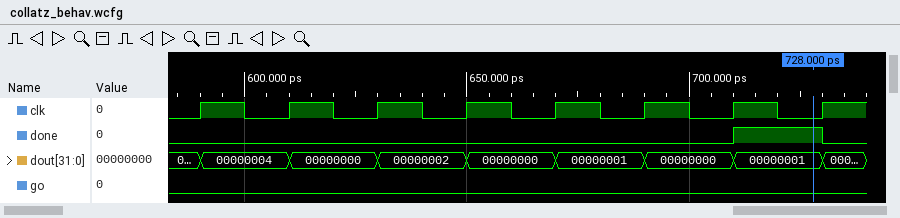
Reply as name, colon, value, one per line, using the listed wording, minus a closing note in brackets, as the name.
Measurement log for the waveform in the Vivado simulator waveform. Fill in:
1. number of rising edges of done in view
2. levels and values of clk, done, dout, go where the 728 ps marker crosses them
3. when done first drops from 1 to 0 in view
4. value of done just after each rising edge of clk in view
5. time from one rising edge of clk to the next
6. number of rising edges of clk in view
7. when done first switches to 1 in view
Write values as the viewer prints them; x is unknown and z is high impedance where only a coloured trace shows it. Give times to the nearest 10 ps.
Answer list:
number of rising edges of done in view: 1
levels and values of clk, done, dout, go where the 728 ps marker crosses them: clk=0, done=1, dout=00000001, go=0
when done first drops from 1 to 0 in view: 730 ps
value of done just after each rising edge of clk in view: 0 0 0 0 0 0 1 0
time from one rising edge of clk to the next: 20 ps
number of rising edges of clk in view: 8
when done first switches to 1 in view: 710 ps
